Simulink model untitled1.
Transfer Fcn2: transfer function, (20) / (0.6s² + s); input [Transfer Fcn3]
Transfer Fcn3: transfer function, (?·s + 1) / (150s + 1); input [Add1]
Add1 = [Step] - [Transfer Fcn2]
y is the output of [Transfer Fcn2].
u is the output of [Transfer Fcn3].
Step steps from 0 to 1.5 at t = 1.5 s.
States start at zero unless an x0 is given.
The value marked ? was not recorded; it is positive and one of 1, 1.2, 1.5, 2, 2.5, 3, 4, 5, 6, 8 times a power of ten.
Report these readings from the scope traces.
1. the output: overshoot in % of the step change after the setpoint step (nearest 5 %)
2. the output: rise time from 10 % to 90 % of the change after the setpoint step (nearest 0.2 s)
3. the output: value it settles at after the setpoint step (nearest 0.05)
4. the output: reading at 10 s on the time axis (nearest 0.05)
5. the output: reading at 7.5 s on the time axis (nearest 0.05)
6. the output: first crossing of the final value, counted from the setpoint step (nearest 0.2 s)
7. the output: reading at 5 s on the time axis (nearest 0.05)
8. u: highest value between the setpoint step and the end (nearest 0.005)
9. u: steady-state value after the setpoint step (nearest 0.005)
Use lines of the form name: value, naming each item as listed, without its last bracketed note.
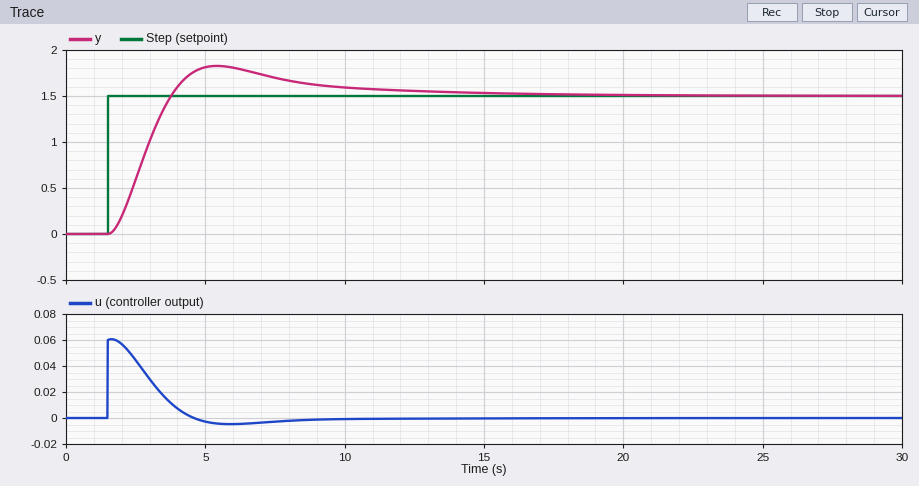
the output: overshoot in % of the step change after the setpoint step: 20 %
the output: rise time from 10 % to 90 % of the change after the setpoint step: 1.6 s
the output: value it settles at after the setpoint step: 1.50
the output: reading at 10 s on the time axis: 1.60
the output: reading at 7.5 s on the time axis: 1.70
the output: first crossing of the final value, counted from the setpoint step: 2.2 s
the output: reading at 5 s on the time axis: 1.80
u: highest value between the setpoint step and the end: 0.060
u: steady-state value after the setpoint step: 0.000
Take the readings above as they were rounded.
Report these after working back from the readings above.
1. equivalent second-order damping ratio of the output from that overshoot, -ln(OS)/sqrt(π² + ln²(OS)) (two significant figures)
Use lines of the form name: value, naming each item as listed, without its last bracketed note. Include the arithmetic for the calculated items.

equivalent second-order damping ratio of the output from that overshoot, -ln(OS)/sqrt(π² + ln²(OS)): ln(0.2) = -1.609; 1.609 / sqrt(9.870 + 2.590) = 0.46
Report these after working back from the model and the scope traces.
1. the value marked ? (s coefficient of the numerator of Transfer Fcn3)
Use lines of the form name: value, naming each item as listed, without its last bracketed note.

the value marked ?: 6
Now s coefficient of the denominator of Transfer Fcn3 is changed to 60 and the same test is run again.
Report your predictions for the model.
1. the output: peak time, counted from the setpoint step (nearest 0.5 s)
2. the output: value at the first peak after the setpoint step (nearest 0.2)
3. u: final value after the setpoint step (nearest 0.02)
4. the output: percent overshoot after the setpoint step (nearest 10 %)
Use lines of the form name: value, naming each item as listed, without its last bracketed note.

the output: peak time, counted from the setpoint step: 2.0 s
the output: value at the first peak after the setpoint step: 2.0
u: final value after the setpoint step: 0.00
the output: percent overshoot after the setpoint step: 30 %
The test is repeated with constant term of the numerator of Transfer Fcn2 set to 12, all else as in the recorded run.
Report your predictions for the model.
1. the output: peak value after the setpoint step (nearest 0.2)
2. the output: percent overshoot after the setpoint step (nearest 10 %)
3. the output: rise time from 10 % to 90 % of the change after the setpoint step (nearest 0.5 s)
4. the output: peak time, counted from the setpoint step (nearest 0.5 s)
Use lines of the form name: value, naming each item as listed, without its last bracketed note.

the output: peak value after the setpoint step: 1.8
the output: percent overshoot after the setpoint step: 20 %
the output: rise time from 10 % to 90 % of the change after the setpoint step: 2.5 s
the output: peak time, counted from the setpoint step: 6.5 s
